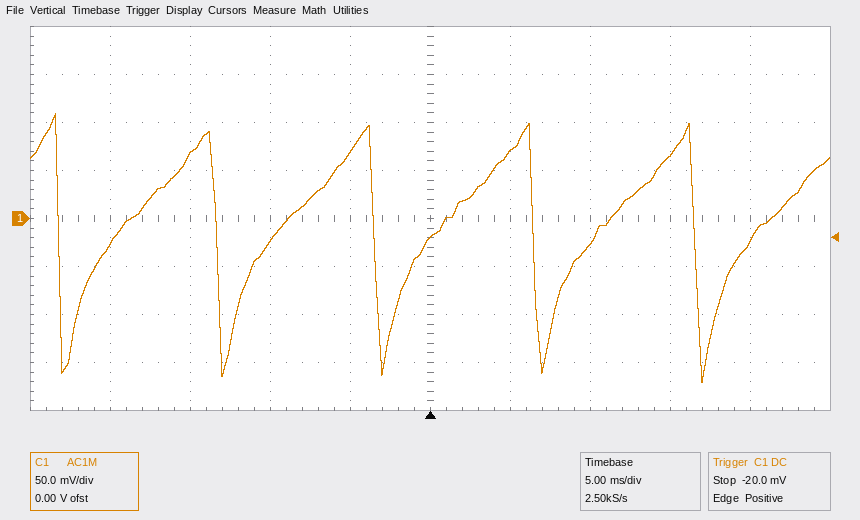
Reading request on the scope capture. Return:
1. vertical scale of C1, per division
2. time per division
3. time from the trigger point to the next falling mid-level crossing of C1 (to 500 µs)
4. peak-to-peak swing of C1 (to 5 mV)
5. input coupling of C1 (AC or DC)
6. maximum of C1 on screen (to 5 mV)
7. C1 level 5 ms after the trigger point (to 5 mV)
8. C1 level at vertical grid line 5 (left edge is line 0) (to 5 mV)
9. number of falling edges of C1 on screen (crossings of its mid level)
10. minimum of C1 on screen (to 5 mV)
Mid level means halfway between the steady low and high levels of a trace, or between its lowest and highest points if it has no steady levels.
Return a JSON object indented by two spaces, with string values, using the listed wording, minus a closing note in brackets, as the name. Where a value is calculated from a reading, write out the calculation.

{
  "vertical scale of C1, per division": "50 mV",
  "time per division": "5 ms",
  "time from the trigger point to the next falling mid-level crossing of C1": "6.5 ms",
  "peak-to-peak swing of C1": "110 mV − (-170 mV) = 280 mV",
  "input coupling of C1": "AC",
  "maximum of C1 on screen": "110 mV",
  "C1 level 5 ms after the trigger point": "70 mV",
  "C1 level at vertical grid line 5 (left edge is line 0)": "-20 mV",
  "number of falling edges of C1 on screen": "5",
  "minimum of C1 on screen": "-170 mV"
}
